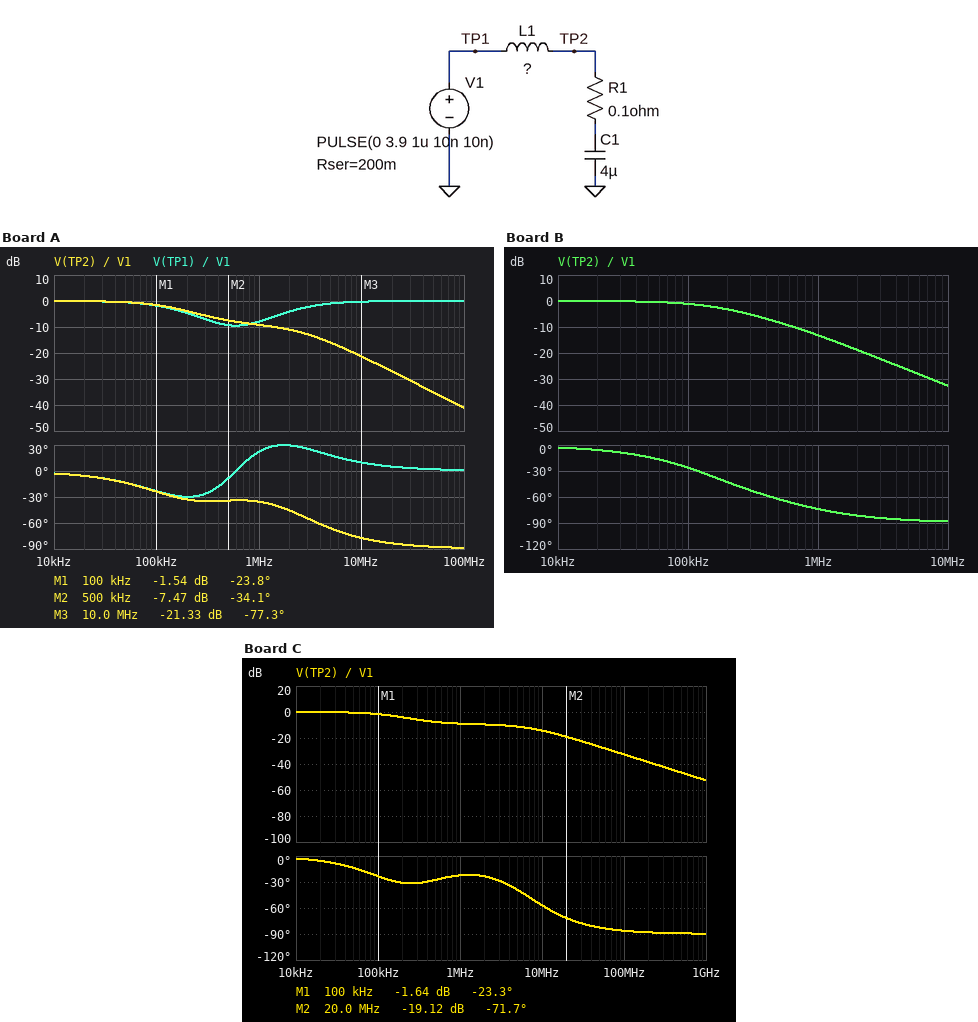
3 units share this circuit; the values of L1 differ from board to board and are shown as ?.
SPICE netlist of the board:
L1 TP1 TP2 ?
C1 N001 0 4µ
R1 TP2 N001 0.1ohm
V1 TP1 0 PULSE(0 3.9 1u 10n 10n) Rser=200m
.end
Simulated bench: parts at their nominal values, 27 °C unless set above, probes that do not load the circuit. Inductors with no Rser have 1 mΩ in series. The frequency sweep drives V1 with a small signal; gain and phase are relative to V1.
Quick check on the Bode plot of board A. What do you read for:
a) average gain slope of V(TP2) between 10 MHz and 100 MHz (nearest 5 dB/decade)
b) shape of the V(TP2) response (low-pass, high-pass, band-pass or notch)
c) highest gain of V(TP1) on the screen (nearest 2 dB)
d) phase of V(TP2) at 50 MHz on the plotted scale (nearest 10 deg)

-20 dB/decade
low-pass
0 dB
-90 deg
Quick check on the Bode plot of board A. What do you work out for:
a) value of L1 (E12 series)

18 nH
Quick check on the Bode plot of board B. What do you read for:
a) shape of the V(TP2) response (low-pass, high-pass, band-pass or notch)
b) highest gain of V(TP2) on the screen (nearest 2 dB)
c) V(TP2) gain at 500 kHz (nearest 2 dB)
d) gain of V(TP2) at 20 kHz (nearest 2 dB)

low-pass
0 dB
-8 dB
0 dB
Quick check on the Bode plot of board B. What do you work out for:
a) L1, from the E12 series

68 nH
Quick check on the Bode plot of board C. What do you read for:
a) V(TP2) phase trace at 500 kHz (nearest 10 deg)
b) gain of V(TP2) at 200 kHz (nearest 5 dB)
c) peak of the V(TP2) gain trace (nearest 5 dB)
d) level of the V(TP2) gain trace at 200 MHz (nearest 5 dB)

-30 deg
-5 dB
0 dB
-40 dB
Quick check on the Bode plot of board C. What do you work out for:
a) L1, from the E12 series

6.8 nH
